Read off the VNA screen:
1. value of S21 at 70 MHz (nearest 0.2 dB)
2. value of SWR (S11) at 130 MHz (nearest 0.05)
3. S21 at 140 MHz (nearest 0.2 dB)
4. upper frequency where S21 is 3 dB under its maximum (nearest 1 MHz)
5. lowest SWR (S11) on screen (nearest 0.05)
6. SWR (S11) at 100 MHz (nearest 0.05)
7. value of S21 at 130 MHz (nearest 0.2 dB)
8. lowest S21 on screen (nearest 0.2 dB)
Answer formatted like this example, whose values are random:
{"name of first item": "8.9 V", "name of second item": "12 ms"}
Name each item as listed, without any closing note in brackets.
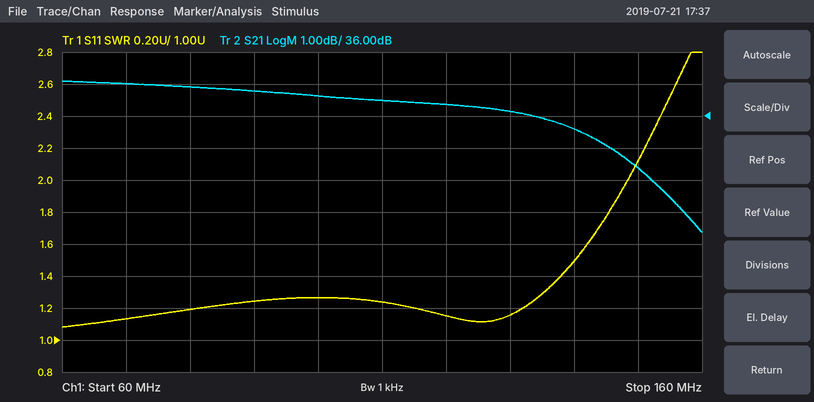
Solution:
{"value of S21 at 70 MHz": "37.0 dB", "value of SWR (S11) at 130 MHz": "1.15", "S21 at 140 MHz": "35.6 dB", "upper frequency where S21 is 3 dB under its maximum": "152 MHz", "lowest SWR (S11) on screen": "1.10", "SWR (S11) at 100 MHz": "1.25", "value of S21 at 130 MHz": "36.2 dB", "lowest S21 on screen": "32.4 dB"}
